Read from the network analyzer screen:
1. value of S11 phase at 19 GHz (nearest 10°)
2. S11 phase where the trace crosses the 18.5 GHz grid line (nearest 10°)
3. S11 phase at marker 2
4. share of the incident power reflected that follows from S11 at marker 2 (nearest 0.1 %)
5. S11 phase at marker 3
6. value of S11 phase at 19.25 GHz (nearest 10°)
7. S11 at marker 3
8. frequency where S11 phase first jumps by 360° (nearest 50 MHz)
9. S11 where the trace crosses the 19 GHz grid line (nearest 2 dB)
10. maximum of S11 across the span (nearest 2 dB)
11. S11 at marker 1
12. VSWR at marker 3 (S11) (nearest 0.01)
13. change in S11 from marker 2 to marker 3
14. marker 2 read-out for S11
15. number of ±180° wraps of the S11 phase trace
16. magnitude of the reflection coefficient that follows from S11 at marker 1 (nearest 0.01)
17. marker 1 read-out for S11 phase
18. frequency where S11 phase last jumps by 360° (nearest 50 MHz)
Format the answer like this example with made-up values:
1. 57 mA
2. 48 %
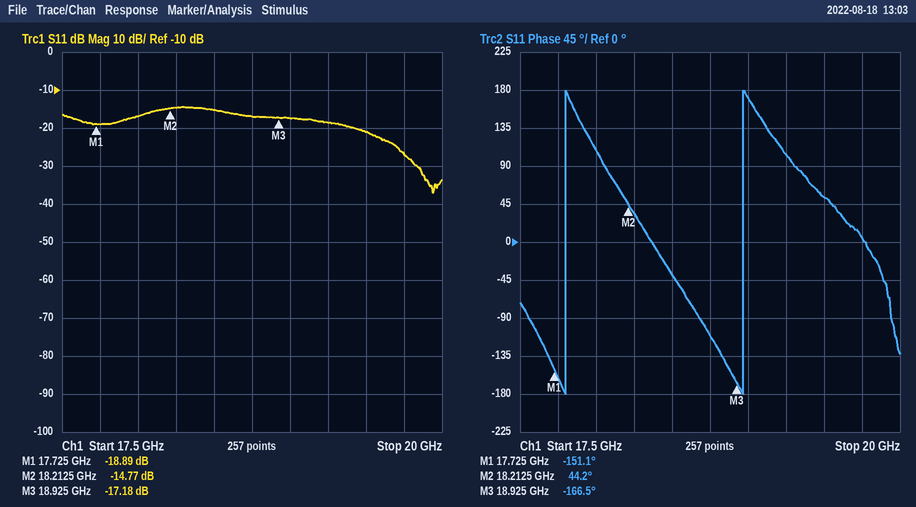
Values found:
1. 170°
2. -40°
3. 44.2°
4. 3.3 %
5. -166.5°
6. 100°
7. -17.18 dB
8. 17.80 GHz
9. -18 dB
10. -14 dB
11. -18.89 dB
12. 1.32
13. -2.41 dB
14. -14.77 dB
15. 2
16. 0.11
17. -151.1°
18. 18.95 GHz
